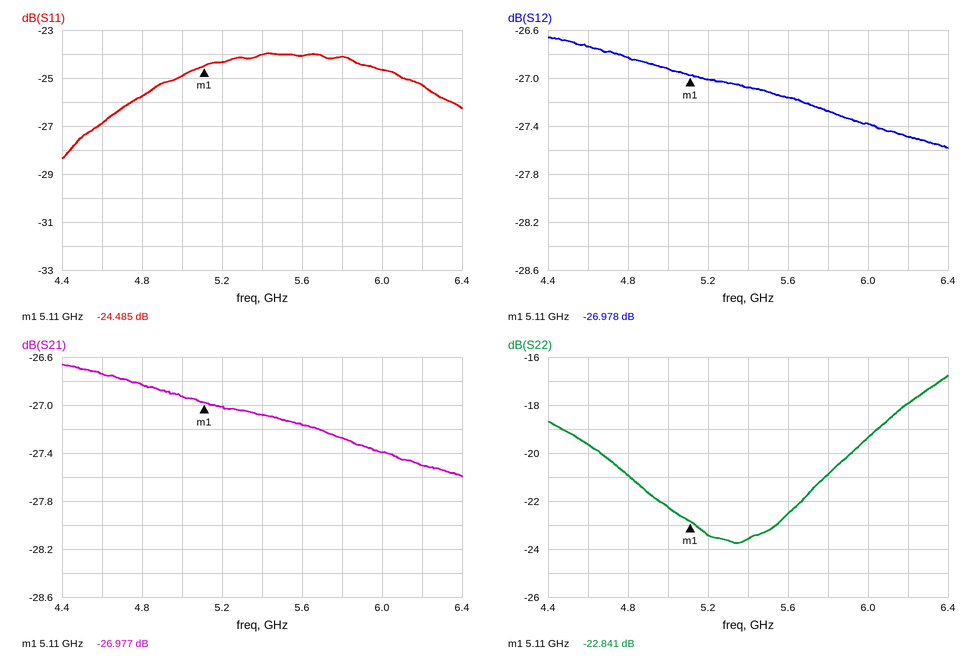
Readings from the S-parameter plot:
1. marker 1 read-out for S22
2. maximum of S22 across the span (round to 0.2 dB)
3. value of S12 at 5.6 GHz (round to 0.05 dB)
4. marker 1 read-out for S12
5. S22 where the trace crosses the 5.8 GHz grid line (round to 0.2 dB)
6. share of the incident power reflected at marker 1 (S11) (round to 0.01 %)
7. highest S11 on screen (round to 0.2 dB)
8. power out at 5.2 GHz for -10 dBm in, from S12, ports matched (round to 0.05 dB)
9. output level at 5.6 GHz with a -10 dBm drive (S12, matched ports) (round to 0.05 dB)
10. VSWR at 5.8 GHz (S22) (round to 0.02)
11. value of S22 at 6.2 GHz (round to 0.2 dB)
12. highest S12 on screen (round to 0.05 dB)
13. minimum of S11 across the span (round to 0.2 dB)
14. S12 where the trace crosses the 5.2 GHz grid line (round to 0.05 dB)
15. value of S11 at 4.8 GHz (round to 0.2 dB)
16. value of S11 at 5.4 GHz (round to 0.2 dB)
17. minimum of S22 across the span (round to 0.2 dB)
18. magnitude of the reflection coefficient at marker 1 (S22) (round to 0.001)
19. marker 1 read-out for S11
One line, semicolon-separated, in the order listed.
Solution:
-22.841 dB; -16.8 dB; -27.15 dB; -26.978 dB; -20.8 dB; 0.36 %; -24.0 dB; -37.00 dBm; -37.15 dBm; 1.20; -18.0 dB; -26.65 dB; -28.4 dB; -27.00 dB; -25.8 dB; -24.0 dB; -23.8 dB; 0.072; -24.485 dB
